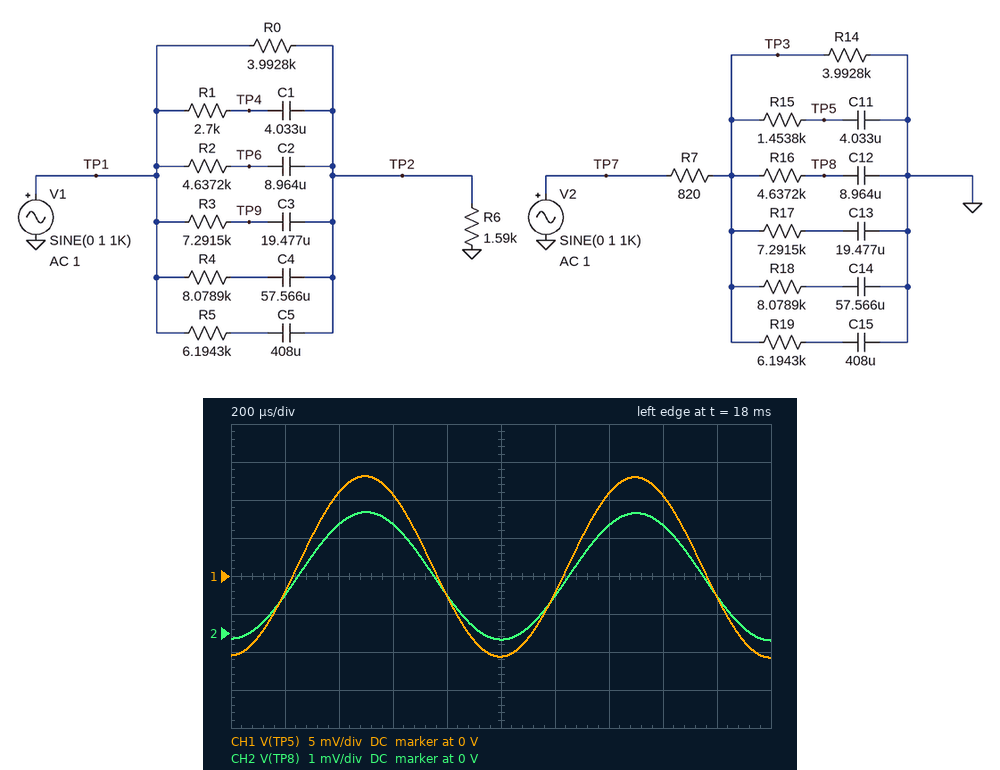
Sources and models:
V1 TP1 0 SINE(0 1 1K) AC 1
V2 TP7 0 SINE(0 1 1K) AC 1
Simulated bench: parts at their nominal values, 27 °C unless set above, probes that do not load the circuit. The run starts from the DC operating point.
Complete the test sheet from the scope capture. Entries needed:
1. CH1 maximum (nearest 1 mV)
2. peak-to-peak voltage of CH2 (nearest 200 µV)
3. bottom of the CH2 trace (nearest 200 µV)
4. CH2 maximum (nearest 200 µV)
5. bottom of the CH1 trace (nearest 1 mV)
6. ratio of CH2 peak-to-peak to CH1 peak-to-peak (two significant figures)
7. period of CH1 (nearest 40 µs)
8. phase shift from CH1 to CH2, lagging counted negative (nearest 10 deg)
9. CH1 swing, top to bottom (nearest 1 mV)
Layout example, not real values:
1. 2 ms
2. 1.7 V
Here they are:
1. 13 mV
2. 3.4 mV
3. -200 µV
4. 3.2 mV
5. -11 mV
6. 0.14
7. 1.00 ms
8. 0 deg
9. 24 mV
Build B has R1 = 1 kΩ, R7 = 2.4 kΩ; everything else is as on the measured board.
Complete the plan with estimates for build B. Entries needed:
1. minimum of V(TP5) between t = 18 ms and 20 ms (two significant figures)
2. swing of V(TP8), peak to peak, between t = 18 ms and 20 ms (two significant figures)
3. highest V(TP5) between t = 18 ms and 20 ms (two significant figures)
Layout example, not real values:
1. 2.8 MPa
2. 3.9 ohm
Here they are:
1. -4.9 mV
2. 1.6 mV
3. 6.6 mV
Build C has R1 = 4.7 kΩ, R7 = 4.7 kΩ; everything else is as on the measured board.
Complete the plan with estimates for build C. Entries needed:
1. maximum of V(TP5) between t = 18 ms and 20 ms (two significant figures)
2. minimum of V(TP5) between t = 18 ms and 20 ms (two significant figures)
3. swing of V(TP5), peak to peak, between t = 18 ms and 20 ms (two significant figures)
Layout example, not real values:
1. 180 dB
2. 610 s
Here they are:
1. 3.8 mV
2. -2.7 mV
3. 6.5 mV
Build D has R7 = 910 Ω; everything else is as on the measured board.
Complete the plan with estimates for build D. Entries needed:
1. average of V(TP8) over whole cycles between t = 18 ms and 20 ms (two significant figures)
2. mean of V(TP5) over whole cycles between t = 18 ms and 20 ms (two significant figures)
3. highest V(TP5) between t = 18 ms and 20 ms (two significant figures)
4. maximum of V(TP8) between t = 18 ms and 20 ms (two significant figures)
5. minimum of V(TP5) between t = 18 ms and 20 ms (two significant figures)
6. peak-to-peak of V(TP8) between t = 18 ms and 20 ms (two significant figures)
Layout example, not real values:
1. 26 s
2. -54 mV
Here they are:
1. 1.4 mV
2. 1.2 mV
3. 12 mV
4. 3.0 mV
5. -10 mV
6. 3.2 mV
